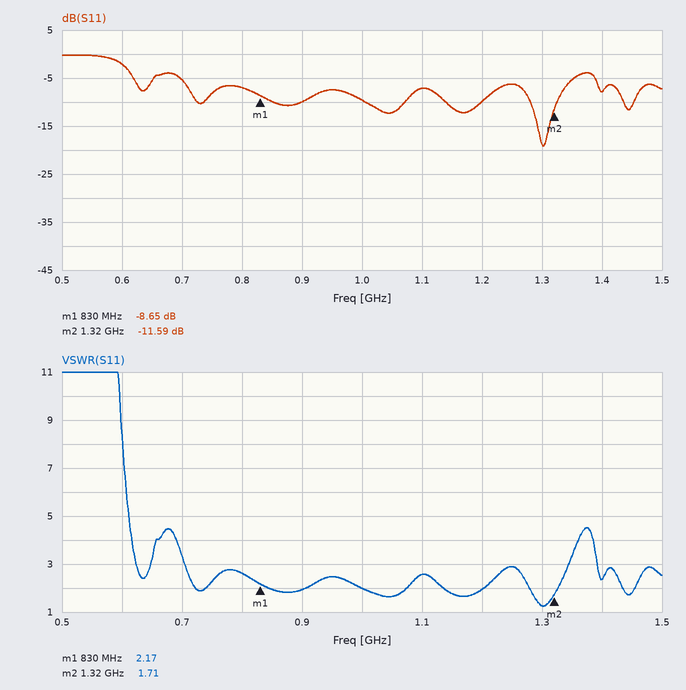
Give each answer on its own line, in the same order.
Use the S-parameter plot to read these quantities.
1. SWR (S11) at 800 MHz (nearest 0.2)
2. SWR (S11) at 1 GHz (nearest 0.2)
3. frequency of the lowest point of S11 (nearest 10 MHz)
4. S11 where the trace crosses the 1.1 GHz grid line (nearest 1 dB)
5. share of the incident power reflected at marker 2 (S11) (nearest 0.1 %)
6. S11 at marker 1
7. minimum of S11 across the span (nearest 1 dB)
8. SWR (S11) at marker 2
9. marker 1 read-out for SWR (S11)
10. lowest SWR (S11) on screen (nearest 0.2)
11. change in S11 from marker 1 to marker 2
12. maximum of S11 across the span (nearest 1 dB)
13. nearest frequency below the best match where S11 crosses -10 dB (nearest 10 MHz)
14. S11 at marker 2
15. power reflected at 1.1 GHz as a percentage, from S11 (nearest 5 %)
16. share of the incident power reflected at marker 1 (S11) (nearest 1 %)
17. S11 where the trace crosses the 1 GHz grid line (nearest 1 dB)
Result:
2.6
2.0
1.30 GHz
-7 dB
6.9 %
-8.65 dB
-19 dB
1.71
2.17
1.2
-2.94 dB
0 dB
1.28 GHz
-11.59 dB
20 %
14 %
-10 dB
